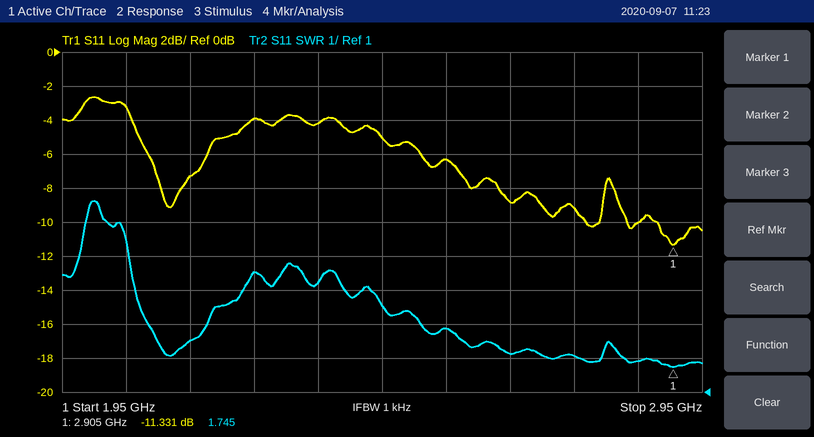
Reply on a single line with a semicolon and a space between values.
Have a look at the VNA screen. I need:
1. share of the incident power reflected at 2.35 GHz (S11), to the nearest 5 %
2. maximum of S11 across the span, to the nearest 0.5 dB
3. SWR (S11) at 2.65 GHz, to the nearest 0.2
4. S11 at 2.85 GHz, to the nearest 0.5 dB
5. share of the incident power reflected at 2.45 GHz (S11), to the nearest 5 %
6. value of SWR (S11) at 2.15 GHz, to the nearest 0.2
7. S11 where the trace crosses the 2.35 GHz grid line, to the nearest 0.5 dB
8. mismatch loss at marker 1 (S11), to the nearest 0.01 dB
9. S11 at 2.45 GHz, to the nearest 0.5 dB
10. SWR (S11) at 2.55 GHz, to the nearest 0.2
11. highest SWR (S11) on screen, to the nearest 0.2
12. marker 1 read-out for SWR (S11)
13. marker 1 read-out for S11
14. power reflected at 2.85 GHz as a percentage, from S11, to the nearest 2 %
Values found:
40 %; -2.5 dB; 2.2; -10.0 dB; 30 %; 2.6; -4.0 dB; 0.33 dB; -5.0 dB; 2.8; 6.6; 1.745; -11.331 dB; 10 %
